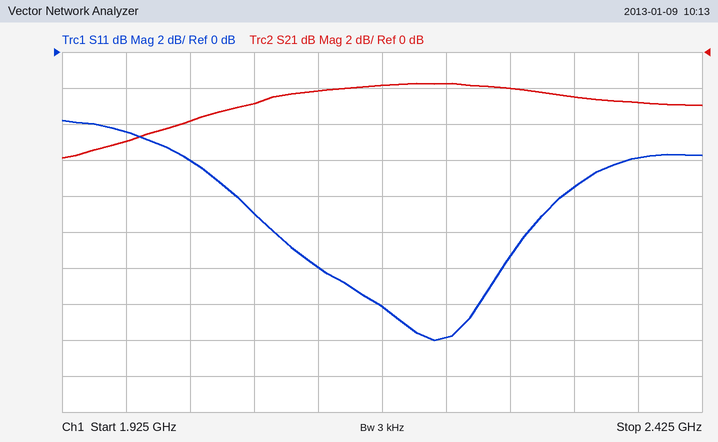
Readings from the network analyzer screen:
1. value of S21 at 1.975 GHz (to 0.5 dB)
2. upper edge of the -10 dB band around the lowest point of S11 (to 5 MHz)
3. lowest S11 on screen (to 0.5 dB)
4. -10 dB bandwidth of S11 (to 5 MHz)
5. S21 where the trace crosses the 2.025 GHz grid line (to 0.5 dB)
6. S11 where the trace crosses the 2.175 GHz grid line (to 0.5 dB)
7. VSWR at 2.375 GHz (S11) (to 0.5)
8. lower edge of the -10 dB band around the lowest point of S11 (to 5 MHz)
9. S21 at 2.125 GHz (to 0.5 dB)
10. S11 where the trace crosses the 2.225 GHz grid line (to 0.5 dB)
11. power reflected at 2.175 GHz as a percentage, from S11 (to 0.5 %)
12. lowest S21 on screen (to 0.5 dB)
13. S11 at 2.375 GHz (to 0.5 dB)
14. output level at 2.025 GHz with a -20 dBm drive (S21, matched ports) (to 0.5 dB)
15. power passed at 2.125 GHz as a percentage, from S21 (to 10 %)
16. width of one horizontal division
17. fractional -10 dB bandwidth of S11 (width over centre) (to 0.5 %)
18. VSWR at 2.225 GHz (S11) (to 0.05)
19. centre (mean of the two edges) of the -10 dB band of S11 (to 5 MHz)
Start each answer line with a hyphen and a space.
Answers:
- -5.0 dB
- 2.290 GHz
- -16.0 dB
- 200 MHz
- -4.0 dB
- -14.0 dB
- 3.0
- 2.090 GHz
- -2.0 dB
- -16.0 dB
- 4.0 %
- -6.0 dB
- -6.0 dB
- -24.0 dBm
- 60 %
- 50 MHz
- 9.0 %
- 1.40
- 2.190 GHz
